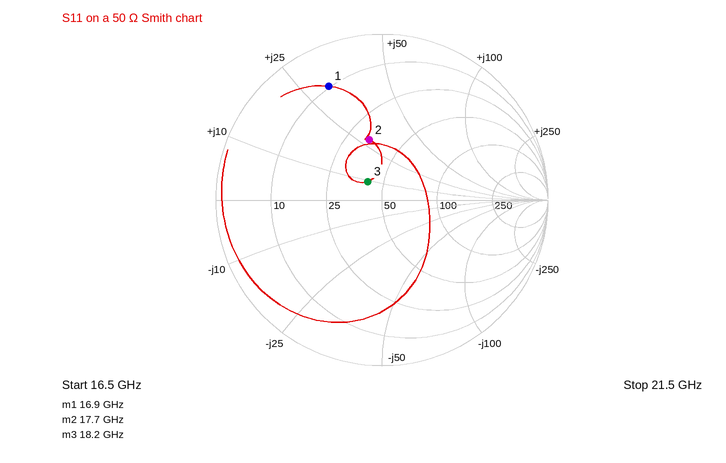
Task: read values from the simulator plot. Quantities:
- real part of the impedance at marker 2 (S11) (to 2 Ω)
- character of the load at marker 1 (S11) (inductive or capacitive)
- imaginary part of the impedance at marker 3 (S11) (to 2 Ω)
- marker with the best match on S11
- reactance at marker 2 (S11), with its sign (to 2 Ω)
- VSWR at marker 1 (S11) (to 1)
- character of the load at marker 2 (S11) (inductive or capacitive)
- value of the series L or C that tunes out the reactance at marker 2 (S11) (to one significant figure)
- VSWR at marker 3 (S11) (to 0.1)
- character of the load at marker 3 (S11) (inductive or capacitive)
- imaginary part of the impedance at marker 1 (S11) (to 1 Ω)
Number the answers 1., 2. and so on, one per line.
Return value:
1. 34 Ω
2. inductive
3. +10 Ω
4. marker 3
5. +28 Ω
6. 7
7. inductive
8. 300 fF
9. 1.3
10. inductive
11. +31 Ω
